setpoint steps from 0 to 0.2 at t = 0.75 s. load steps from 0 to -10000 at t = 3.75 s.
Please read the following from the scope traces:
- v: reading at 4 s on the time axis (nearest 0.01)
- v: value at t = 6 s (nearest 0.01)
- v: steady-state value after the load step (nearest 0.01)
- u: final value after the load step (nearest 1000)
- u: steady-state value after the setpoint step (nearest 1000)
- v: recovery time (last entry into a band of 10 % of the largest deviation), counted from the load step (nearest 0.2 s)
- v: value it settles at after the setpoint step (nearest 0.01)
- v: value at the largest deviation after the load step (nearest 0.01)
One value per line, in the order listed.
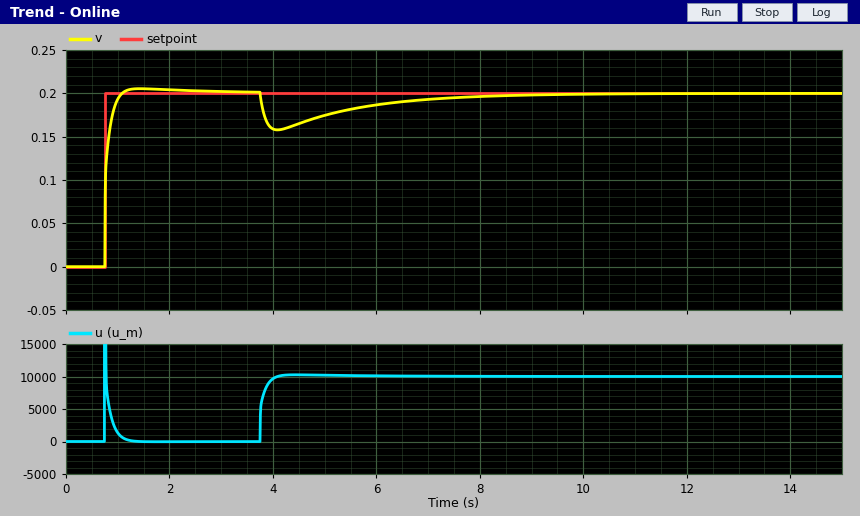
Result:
0.16
0.19
0.20
10000
0
4.0 s
0.20
0.16
